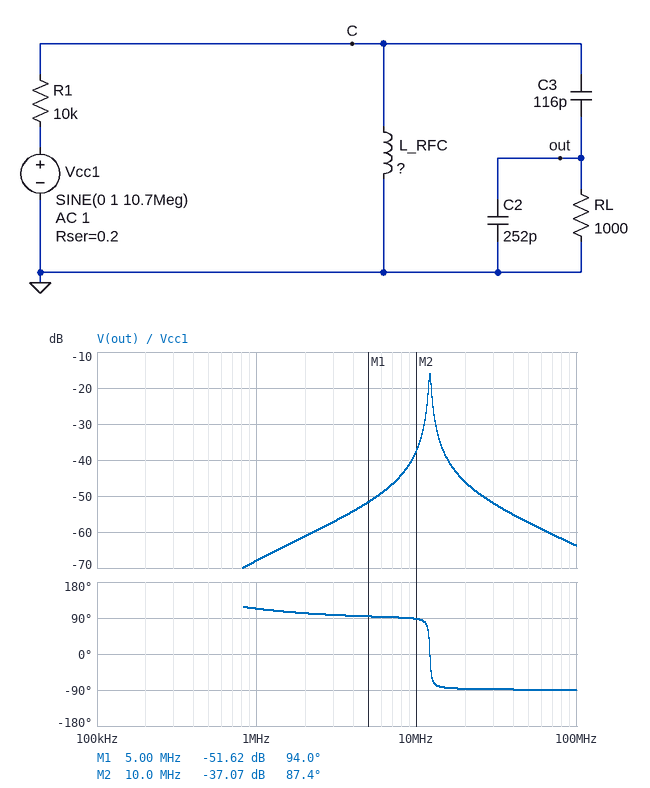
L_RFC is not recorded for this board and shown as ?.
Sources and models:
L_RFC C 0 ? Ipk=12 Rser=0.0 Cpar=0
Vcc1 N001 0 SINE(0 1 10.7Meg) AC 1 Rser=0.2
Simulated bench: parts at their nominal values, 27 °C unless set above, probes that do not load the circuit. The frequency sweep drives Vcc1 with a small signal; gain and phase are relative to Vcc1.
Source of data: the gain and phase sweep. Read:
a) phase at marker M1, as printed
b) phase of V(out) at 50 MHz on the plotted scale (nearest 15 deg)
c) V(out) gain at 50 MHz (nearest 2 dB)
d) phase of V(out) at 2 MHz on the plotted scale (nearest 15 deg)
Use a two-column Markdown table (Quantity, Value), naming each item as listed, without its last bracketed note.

| Quantity | Value |
|---|---|
| phase at marker M1, as printed | 94.0 deg |
| phase of V(out) at 50 MHz on the plotted scale | -90 deg |
| V(out) gain at 50 MHz | -58 dB |
| phase of V(out) at 2 MHz on the plotted scale | 105 deg |
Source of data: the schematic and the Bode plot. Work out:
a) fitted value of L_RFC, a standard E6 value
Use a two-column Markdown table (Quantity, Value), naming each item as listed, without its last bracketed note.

| Quantity | Value |
|---|---|
| fitted value of L_RFC, a standard E6 value | 2.2 µH |
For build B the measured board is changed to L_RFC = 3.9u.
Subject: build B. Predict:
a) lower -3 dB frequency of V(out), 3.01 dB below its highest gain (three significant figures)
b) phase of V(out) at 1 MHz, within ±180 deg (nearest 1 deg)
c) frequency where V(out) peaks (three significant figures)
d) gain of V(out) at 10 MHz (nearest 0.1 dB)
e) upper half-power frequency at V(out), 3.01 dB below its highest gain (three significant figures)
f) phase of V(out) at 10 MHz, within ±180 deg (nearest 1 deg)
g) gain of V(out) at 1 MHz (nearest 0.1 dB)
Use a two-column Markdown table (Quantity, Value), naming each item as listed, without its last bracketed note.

| Quantity | Value |
|---|---|
| lower -3 dB frequency of V(out), 3.01 dB below its highest gain | 8.84 MHz |
| phase of V(out) at 1 MHz, within ±180 deg | 113 deg |
| frequency where V(out) peaks | 9.04 MHz |
| gain of V(out) at 10 MHz | -29.5 dB |
| upper half-power frequency at V(out), 3.01 dB below its highest gain | 9.24 MHz |
| phase of V(out) at 10 MHz, within ±180 deg | -75 deg |
| gain of V(out) at 1 MHz | -62.9 dB |
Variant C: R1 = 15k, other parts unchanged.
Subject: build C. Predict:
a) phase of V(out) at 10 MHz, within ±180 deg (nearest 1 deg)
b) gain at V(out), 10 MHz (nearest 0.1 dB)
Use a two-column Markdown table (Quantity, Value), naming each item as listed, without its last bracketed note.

| Quantity | Value |
|---|---|
| phase of V(out) at 10 MHz, within ±180 deg | 88 deg |
| gain at V(out), 10 MHz | -40.6 dB |
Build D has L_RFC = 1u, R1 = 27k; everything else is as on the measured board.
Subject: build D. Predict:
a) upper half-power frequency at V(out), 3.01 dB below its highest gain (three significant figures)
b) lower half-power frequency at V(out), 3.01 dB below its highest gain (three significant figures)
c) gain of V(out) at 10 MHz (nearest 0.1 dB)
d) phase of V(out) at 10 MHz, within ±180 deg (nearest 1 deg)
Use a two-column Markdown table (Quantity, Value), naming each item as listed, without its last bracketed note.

| Quantity | Value |
|---|---|
| upper half-power frequency at V(out), 3.01 dB below its highest gain | 18.0 MHz |
| lower half-power frequency at V(out), 3.01 dB below its highest gain | 17.7 MHz |
| gain of V(out) at 10 MHz | -59.4 dB |
| phase of V(out) at 10 MHz, within ±180 deg | 92 deg |
